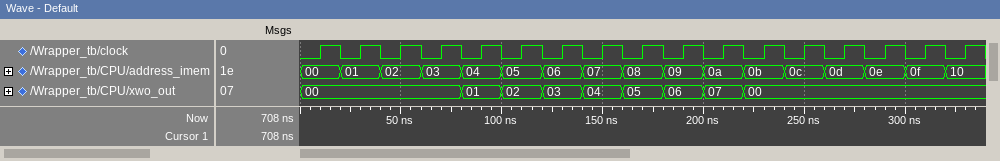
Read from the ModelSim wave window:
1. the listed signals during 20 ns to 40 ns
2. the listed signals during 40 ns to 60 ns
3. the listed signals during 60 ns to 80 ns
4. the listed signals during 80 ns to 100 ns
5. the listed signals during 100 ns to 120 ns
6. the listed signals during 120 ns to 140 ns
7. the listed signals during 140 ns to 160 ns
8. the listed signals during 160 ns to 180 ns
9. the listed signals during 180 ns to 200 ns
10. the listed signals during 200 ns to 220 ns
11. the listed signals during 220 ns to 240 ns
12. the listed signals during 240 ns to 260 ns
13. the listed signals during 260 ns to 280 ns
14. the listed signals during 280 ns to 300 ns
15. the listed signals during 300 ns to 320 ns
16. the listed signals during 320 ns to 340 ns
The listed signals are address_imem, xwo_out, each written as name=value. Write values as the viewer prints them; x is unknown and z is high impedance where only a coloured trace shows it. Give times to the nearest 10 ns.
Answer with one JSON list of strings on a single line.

["address_imem=01, xwo_out=00", "address_imem=02, xwo_out=00", "address_imem=03, xwo_out=00", "address_imem=04, xwo_out=01", "address_imem=05, xwo_out=02", "address_imem=06, xwo_out=03", "address_imem=07, xwo_out=04", "address_imem=08, xwo_out=05", "address_imem=09, xwo_out=06", "address_imem=0a, xwo_out=07", "address_imem=0b, xwo_out=00", "address_imem=0c, xwo_out=00", "address_imem=0d, xwo_out=00", "address_imem=0e, xwo_out=00", "address_imem=0f, xwo_out=00", "address_imem=10, xwo_out=00"]
